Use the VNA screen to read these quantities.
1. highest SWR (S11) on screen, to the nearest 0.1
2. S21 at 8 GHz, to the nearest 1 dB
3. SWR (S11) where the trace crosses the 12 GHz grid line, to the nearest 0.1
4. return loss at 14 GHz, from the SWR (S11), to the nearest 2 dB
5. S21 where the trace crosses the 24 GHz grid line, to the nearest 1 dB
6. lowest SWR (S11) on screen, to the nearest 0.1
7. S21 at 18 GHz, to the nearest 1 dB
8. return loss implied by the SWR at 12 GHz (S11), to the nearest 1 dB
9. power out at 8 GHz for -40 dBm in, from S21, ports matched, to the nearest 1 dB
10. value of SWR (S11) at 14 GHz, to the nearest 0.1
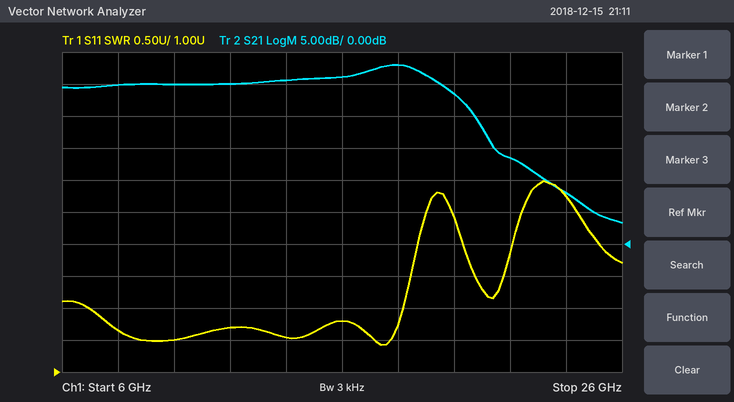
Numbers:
4.0
25 dB
1.7
14 dB
8 dB
1.4
28 dB
12 dB
-15 dBm
1.5
